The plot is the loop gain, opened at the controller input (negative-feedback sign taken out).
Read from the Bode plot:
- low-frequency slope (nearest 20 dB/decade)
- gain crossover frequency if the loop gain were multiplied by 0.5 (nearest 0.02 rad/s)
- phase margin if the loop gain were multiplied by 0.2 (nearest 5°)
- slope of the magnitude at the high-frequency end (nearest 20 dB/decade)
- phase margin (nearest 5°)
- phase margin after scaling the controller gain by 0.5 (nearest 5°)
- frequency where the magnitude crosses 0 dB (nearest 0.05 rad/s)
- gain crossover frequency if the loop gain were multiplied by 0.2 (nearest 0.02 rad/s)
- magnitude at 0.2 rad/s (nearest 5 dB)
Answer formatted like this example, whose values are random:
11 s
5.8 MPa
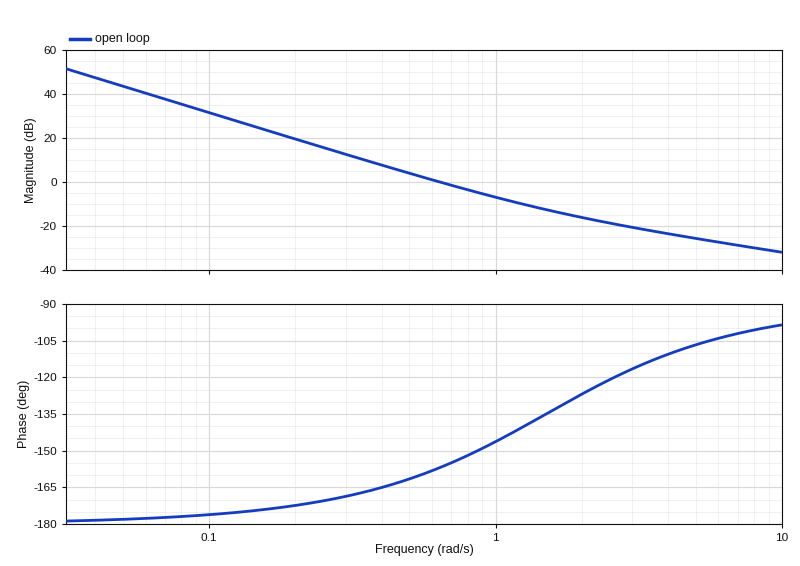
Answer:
-40 dB/decade
0.44 rad/s
10°
-20 dB/decade
25°
15°
0.65 rad/s
0.28 rad/s
20 dB
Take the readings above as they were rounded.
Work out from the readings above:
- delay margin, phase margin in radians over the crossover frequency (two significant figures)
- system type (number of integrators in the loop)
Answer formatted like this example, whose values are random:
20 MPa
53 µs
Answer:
0.67 s
2
